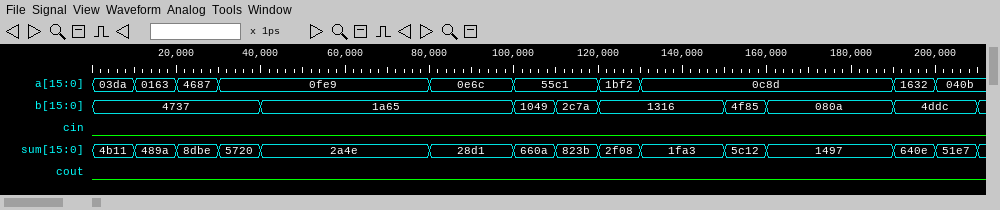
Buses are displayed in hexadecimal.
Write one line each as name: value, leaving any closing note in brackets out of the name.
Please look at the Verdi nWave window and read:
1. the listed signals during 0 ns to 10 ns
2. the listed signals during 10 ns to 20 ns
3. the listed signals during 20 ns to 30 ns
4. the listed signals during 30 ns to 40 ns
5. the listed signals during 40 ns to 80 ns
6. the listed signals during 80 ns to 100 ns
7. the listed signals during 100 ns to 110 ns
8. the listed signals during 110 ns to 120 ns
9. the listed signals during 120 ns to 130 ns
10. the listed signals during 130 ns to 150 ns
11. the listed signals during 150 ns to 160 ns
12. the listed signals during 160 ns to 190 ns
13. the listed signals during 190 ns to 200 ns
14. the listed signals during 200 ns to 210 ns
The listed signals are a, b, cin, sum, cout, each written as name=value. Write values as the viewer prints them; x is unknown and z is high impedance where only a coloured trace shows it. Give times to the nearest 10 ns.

the listed signals during 0 ns to 10 ns: a=03da, b=4737, cin=0, sum=4b11, cout=0
the listed signals during 10 ns to 20 ns: a=0163, b=4737, cin=0, sum=489a, cout=0
the listed signals during 20 ns to 30 ns: a=4687, b=4737, cin=0, sum=8dbe, cout=0
the listed signals during 30 ns to 40 ns: a=0fe9, b=4737, cin=0, sum=5720, cout=0
the listed signals during 40 ns to 80 ns: a=0fe9, b=1a65, cin=0, sum=2a4e, cout=0
the listed signals during 80 ns to 100 ns: a=0e6c, b=1a65, cin=0, sum=28d1, cout=0
the listed signals during 100 ns to 110 ns: a=55c1, b=1049, cin=0, sum=660a, cout=0
the listed signals during 110 ns to 120 ns: a=55c1, b=2c7a, cin=0, sum=823b, cout=0
the listed signals during 120 ns to 130 ns: a=1bf2, b=1316, cin=0, sum=2f08, cout=0
the listed signals during 130 ns to 150 ns: a=0c8d, b=1316, cin=0, sum=1fa3, cout=0
the listed signals during 150 ns to 160 ns: a=0c8d, b=4f85, cin=0, sum=5c12, cout=0
the listed signals during 160 ns to 190 ns: a=0c8d, b=080a, cin=0, sum=1497, cout=0
the listed signals during 190 ns to 200 ns: a=1632, b=4ddc, cin=0, sum=640e, cout=0
the listed signals during 200 ns to 210 ns: a=040b, b=4ddc, cin=0, sum=51e7, cout=0
